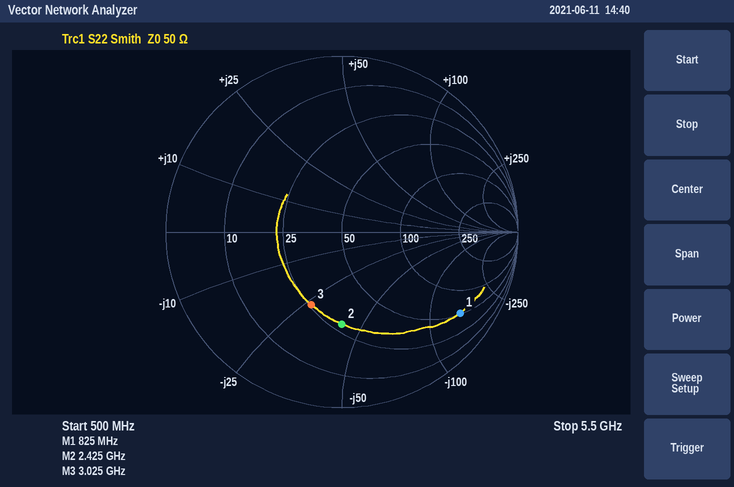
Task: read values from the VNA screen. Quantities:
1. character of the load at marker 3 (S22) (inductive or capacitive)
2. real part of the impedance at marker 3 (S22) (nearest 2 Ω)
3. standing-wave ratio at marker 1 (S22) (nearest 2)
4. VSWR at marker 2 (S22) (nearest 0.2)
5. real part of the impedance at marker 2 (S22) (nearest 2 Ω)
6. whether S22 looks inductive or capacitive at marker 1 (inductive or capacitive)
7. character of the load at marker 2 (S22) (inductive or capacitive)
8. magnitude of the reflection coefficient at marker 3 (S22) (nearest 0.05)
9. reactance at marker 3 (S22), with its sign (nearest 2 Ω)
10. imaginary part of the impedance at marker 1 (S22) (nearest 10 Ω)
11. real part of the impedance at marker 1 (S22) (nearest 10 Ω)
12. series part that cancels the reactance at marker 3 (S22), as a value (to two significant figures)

capacitive
26 Ω
10
3.2
28 Ω
capacitive
capacitive
0.45
-26 Ω
-140 Ω
50 Ω
1.4 nH
